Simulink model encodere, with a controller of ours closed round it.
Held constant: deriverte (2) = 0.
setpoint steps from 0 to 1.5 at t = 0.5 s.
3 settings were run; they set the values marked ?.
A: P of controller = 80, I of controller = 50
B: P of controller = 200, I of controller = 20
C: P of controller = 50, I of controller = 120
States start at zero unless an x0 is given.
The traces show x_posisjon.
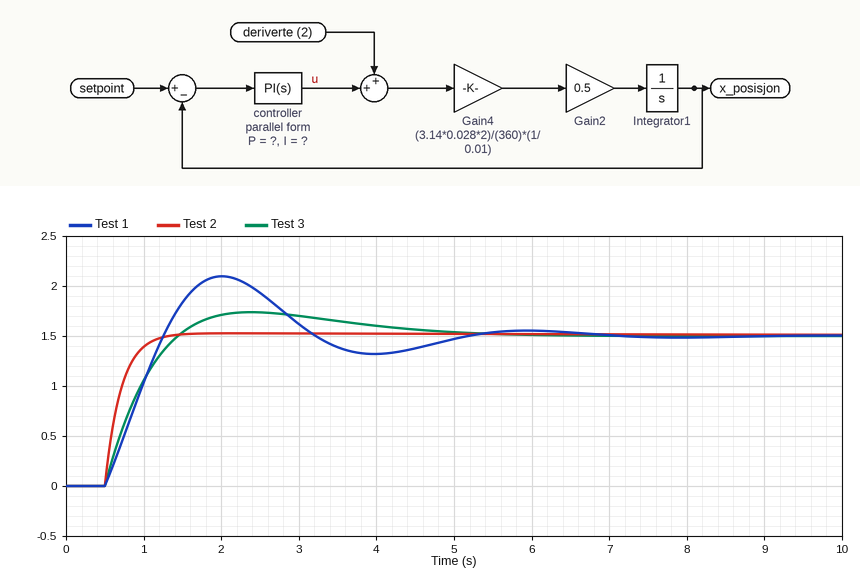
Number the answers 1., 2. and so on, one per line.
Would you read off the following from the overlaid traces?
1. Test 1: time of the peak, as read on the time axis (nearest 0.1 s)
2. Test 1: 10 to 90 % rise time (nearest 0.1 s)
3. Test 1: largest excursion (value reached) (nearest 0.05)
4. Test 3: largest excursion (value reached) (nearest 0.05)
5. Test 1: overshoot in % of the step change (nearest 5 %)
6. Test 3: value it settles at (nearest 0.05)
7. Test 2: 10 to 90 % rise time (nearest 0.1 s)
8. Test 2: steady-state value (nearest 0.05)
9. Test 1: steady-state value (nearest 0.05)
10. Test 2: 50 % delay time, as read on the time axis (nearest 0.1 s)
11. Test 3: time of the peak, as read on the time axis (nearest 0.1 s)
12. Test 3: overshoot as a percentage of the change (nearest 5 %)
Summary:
1. 2.0 s
2. 0.6 s
3. 2.10
4. 1.75
5. 40 %
6. 1.50
7. 0.4 s
8. 1.50
9. 1.50
10. 0.6 s
11. 2.4 s
12. 15 %
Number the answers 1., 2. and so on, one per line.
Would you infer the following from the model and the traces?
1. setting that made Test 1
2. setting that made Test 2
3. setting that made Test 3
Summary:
1. C
2. B
3. A
